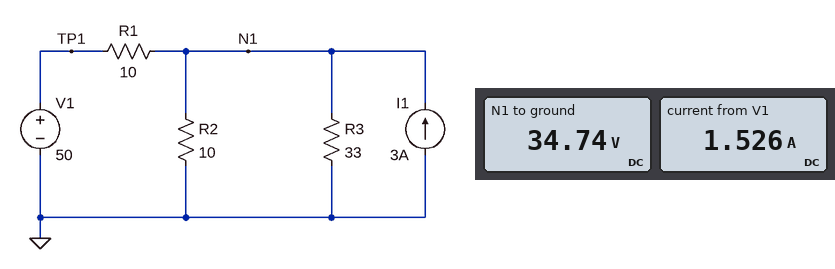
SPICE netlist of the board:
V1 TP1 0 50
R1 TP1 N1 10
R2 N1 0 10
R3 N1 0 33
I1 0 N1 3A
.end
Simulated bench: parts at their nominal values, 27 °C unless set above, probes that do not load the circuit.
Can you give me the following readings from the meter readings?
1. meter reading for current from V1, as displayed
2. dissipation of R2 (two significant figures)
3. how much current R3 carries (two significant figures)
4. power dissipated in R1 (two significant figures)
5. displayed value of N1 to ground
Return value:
1.526 A
120 W
1.1 A
23 W
34.74 V
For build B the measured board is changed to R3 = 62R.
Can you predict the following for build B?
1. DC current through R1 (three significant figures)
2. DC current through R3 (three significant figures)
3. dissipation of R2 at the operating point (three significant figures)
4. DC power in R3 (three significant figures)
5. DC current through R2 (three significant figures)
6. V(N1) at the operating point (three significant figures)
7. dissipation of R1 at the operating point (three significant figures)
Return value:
1.30 A
597 mA
137 W
22.1 W
3.70 A
37.0 V
16.9 W
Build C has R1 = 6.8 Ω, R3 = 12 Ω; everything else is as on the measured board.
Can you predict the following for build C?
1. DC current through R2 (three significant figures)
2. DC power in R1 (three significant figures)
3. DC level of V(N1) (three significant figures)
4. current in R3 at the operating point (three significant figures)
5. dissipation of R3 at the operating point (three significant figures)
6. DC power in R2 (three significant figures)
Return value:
3.13 A
51.2 W
31.3 V
2.61 A
81.8 W
98.2 W
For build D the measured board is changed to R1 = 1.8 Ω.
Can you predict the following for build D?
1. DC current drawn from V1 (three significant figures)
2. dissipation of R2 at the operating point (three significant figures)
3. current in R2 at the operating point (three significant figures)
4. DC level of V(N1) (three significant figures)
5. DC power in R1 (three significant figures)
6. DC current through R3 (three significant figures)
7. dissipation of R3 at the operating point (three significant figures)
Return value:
2.85 A
201 W
4.49 A
44.9 V
14.6 W
1.36 A
61.0 W
